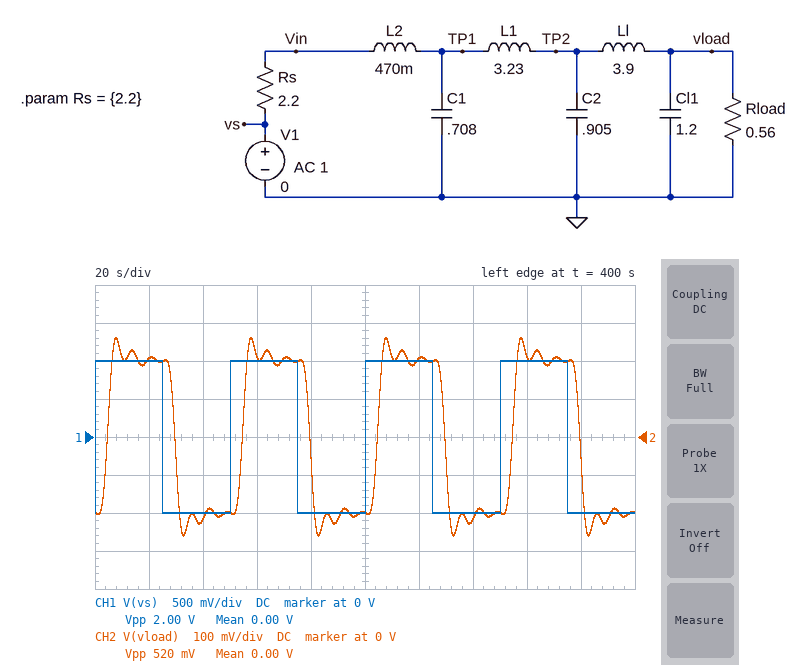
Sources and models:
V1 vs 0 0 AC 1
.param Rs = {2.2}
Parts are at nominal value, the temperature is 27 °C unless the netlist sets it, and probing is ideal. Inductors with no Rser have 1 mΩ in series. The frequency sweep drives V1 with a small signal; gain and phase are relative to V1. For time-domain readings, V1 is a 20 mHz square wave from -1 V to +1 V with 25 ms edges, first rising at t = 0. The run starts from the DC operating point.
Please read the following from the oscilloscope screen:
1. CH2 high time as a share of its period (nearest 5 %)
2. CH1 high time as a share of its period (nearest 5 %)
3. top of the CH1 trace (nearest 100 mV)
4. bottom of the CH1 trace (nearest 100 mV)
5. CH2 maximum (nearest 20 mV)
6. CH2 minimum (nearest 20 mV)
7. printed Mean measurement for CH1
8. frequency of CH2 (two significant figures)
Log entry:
50 %
50 %
1.0 V
-1.0 V
260 mV
-260 mV
0.00 V
20 mHz
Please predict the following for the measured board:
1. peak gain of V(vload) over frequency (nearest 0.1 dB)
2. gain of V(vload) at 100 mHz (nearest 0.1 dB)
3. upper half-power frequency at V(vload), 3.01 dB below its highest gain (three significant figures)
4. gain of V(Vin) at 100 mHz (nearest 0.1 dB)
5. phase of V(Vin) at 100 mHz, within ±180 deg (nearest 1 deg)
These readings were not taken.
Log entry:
-13.4 dB
-15.5 dB
151 mHz
-6.9 dB
-46 deg
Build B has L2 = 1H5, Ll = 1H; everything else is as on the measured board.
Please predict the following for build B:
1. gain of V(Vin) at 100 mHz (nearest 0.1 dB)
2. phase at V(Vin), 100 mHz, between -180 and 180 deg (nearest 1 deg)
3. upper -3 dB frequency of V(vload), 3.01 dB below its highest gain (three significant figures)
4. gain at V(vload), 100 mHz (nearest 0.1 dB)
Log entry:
-2.3 dB
-4 deg
223 mHz
-13.5 dB
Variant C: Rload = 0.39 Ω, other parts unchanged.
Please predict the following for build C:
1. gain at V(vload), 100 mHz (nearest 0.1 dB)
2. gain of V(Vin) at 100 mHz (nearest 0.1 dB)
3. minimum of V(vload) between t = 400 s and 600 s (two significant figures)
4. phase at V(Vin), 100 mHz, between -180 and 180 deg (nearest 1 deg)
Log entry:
-18.2 dB
-7.0 dB
-190 mV
-50 deg
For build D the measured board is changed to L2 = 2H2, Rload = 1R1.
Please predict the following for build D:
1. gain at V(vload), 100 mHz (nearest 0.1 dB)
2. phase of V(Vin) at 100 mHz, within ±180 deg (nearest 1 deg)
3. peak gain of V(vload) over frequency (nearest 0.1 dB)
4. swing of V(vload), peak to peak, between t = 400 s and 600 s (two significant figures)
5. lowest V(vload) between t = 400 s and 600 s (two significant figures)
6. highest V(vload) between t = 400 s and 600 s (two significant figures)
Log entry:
-10.2 dB
-17 deg
-9.5 dB
840 mV
-420 mV
420 mV
